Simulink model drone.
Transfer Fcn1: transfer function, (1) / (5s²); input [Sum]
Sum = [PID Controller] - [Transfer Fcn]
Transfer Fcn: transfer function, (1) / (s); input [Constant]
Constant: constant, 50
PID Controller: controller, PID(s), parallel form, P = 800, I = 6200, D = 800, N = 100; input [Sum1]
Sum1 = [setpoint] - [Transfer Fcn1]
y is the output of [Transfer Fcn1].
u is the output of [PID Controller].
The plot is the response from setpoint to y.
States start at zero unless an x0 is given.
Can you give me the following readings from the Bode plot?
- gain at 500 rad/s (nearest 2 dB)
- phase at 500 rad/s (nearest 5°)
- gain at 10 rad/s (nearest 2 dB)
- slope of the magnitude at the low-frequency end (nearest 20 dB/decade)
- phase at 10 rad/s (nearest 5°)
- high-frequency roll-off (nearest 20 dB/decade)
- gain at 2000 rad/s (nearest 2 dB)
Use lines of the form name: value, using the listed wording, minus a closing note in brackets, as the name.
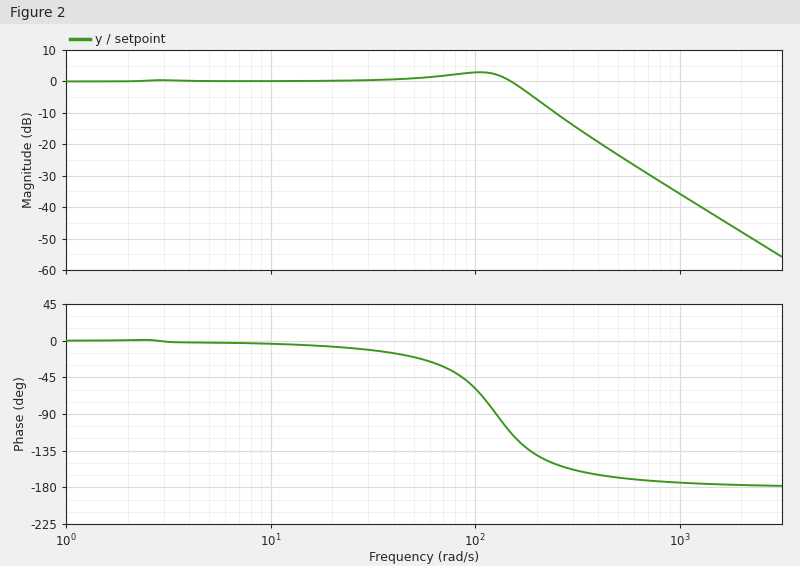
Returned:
gain at 500 rad/s: -24 dB
phase at 500 rad/s: -170°
gain at 10 rad/s: 0 dB
slope of the magnitude at the low-frequency end: 0 dB/decade
phase at 10 rad/s: -5°
high-frequency roll-off: -40 dB/decade
gain at 2000 rad/s: -48 dB
